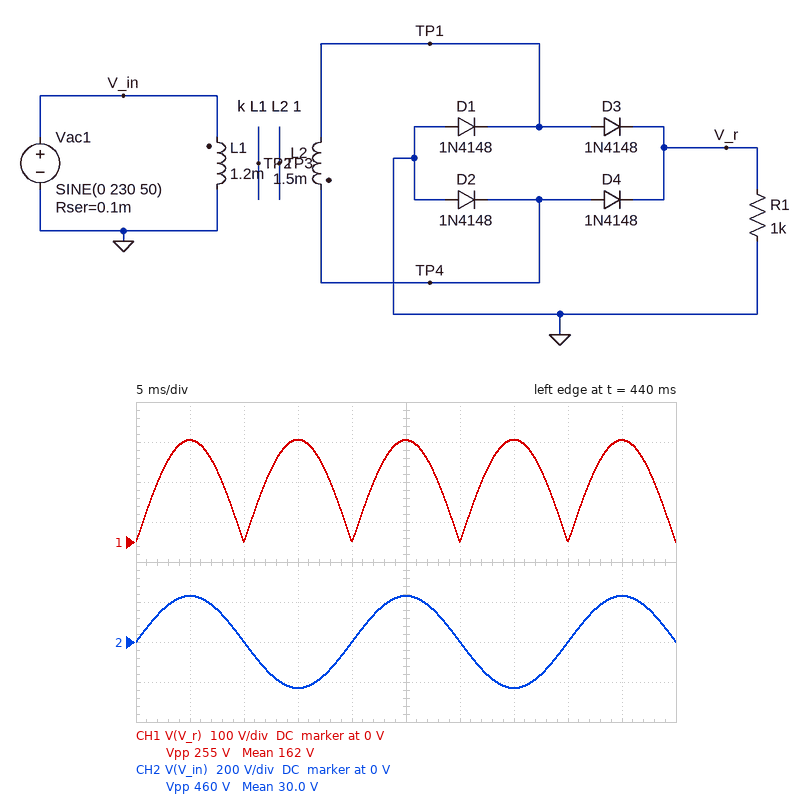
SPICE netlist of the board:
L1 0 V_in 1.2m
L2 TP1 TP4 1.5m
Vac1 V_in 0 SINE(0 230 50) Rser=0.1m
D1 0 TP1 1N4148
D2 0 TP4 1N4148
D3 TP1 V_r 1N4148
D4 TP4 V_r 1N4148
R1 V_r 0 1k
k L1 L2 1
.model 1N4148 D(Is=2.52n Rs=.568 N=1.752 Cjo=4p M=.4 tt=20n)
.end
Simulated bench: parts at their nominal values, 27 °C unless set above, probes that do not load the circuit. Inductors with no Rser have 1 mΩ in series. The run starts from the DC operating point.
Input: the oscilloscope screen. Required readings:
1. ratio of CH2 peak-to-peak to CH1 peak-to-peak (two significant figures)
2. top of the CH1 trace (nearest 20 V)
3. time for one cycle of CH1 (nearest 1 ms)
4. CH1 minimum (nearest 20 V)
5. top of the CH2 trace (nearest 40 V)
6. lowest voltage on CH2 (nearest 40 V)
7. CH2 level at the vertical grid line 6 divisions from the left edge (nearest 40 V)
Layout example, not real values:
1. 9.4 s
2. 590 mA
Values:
1. 1.8
2. 260 V
3. 10 ms
4. 0 V
5. 240 V
6. -240 V
7. 0 V
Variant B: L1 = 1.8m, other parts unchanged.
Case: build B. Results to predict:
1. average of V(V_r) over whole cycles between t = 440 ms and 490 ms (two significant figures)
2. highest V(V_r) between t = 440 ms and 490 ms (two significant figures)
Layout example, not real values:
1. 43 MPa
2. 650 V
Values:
1. 130 V
2. 210 V
